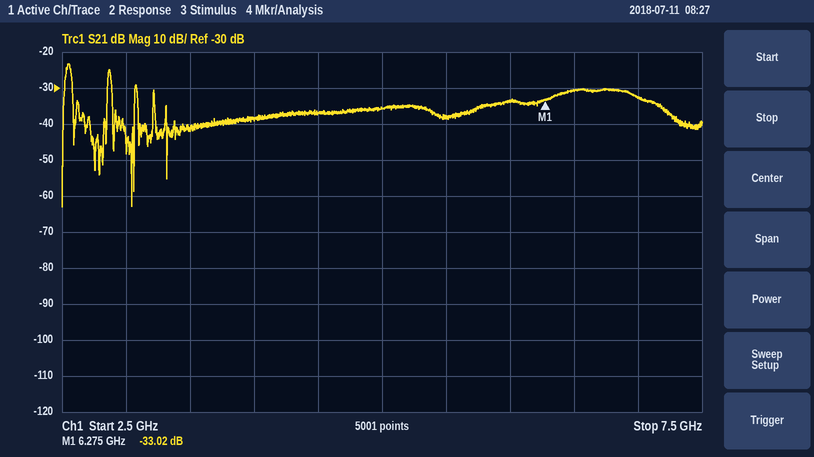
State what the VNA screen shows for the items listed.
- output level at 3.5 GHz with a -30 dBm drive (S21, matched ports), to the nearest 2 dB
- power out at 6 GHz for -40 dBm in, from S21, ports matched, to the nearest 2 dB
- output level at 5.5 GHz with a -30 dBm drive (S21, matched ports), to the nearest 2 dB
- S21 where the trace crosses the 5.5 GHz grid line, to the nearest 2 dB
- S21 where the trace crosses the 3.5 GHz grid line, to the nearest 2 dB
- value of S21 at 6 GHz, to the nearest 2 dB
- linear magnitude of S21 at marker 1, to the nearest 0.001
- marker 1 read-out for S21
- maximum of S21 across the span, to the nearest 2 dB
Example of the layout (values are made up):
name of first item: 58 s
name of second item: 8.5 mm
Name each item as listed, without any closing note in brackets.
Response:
output level at 3.5 GHz with a -30 dBm drive (S21, matched ports), to the nearest 2 dB: -72 dBm
power out at 6 GHz for -40 dBm in, from S21, ports matched, to the nearest 2 dB: -74 dBm
output level at 5.5 GHz with a -30 dBm drive (S21, matched ports), to the nearest 2 dB: -68 dBm
S21 where the trace crosses the 5.5 GHz grid line, to the nearest 2 dB: -38 dB
S21 where the trace crosses the 3.5 GHz grid line, to the nearest 2 dB: -42 dB
value of S21 at 6 GHz, to the nearest 2 dB: -34 dB
linear magnitude of S21 at marker 1, to the nearest 0.001: 0.022
marker 1 read-out for S21: -33.02 dB
maximum of S21 across the span, to the nearest 2 dB: -24 dB
